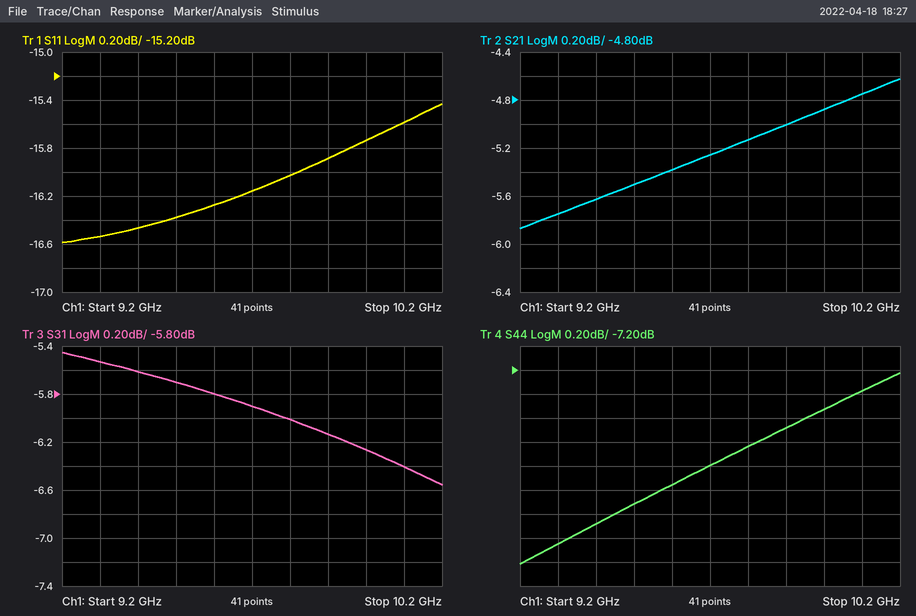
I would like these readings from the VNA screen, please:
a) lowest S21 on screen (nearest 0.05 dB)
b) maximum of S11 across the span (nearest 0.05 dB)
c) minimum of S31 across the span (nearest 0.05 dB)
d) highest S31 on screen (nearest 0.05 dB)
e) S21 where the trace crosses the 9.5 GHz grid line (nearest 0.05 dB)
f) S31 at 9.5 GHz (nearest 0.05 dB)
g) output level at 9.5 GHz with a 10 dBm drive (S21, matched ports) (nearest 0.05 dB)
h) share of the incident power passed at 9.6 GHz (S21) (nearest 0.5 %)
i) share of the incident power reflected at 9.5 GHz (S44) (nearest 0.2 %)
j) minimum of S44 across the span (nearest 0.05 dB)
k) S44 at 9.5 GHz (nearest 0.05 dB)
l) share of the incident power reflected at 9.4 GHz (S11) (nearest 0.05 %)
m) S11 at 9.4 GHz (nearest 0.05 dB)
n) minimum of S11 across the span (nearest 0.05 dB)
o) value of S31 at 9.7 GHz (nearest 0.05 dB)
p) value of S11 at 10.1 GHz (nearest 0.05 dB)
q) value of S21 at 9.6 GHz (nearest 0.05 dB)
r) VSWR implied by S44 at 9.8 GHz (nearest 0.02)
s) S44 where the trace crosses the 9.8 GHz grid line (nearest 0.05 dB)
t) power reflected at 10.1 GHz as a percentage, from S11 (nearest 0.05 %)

-5.85 dB
-15.45 dB
-6.55 dB
-5.45 dB
-5.50 dB
-5.70 dB
4.50 dBm
29.0 %
14.8 %
-8.80 dB
-8.30 dB
2.25 %
-16.45 dB
-16.60 dB
-5.90 dB
-15.60 dB
-5.40 dB
2.36
-7.85 dB
2.75 %
